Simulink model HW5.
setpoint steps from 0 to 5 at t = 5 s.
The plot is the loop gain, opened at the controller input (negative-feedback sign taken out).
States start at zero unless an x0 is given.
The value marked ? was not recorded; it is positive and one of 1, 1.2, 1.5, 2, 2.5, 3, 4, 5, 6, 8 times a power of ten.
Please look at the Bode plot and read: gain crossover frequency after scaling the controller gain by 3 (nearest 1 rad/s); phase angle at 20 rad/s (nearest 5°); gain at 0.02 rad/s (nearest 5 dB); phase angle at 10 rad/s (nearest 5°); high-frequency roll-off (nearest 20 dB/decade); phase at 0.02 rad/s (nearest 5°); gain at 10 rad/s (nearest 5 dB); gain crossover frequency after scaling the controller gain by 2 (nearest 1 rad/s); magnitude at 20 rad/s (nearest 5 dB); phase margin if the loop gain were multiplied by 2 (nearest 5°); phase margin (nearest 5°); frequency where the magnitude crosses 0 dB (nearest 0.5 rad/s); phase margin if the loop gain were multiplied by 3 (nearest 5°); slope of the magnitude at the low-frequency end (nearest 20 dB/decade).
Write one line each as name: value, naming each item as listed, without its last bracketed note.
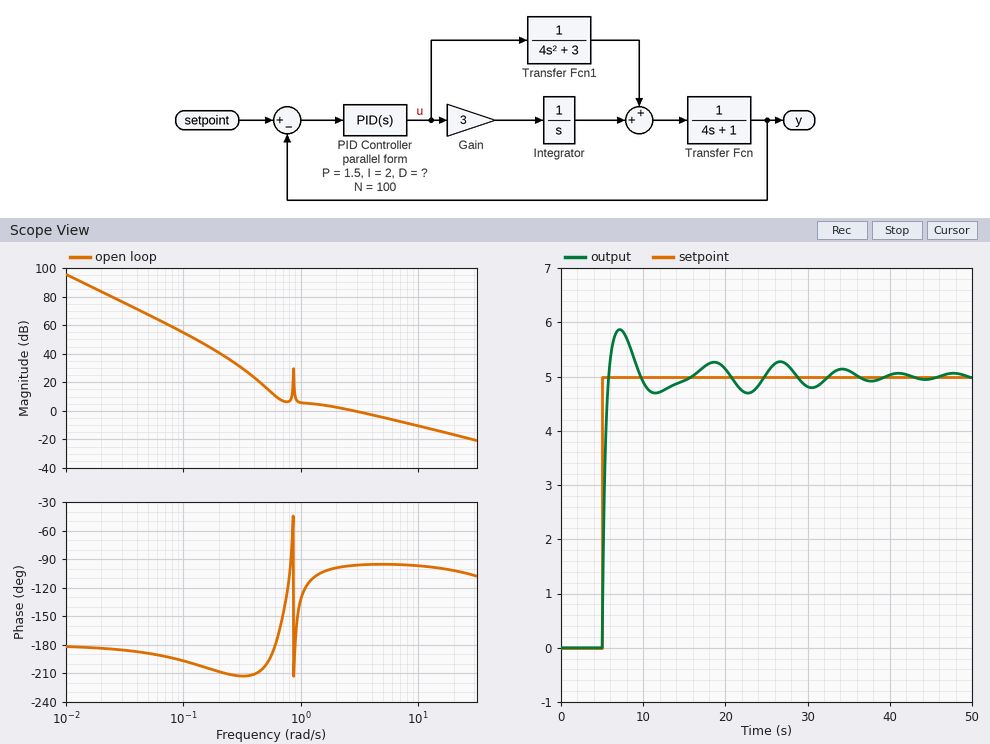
gain crossover frequency after scaling the controller gain by 3: 9 rad/s
phase angle at 20 rad/s: -100°
gain at 0.02 rad/s: 85 dB
phase angle at 10 rad/s: -95°
high-frequency roll-off: -20 dB/decade
phase at 0.02 rad/s: -185°
gain at 10 rad/s: -10 dB
gain crossover frequency after scaling the controller gain by 2: 6 rad/s
magnitude at 20 rad/s: -15 dB
phase margin if the loop gain were multiplied by 2: 85°
phase margin: 85°
frequency where the magnitude crosses 0 dB: 3.0 rad/s
phase margin if the loop gain were multiplied by 3: 85°
slope of the magnitude at the low-frequency end: -40 dB/decade
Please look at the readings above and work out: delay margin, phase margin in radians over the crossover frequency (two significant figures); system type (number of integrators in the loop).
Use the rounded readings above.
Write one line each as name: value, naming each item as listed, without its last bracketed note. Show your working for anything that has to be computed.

delay margin, phase margin in radians over the crossover frequency: 85 × π / 180 / 3 = 0.49 s
system type: 2
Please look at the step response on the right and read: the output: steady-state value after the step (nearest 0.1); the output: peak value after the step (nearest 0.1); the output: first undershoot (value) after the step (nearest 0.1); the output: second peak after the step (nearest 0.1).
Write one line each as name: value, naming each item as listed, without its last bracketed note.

the output: steady-state value after the step: 5.0
the output: peak value after the step: 5.9
the output: first undershoot (value) after the step: 4.7
the output: second peak after the step: 5.3
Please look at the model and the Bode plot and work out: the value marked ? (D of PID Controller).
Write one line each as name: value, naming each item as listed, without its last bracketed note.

the value marked ?: 4
